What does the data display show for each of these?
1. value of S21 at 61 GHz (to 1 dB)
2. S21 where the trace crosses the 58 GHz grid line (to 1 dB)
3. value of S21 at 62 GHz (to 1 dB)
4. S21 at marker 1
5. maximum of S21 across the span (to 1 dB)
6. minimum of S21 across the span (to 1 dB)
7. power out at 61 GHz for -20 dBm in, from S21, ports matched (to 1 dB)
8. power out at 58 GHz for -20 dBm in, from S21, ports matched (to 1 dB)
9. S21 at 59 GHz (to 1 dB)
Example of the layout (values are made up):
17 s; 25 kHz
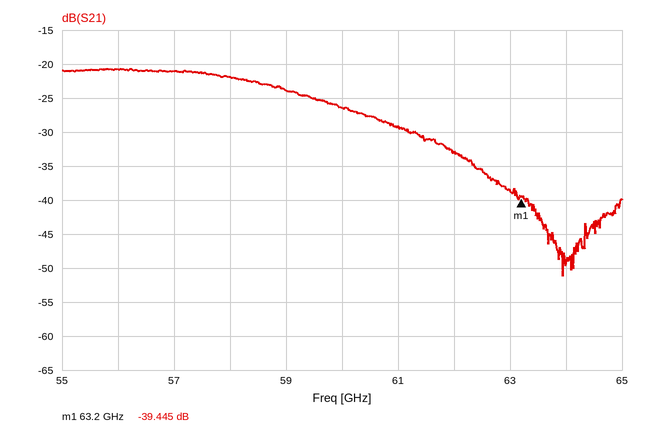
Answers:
-29 dB; -22 dB; -33 dB; -39.445 dB; -21 dB; -51 dB; -49 dBm; -42 dBm; -24 dB
